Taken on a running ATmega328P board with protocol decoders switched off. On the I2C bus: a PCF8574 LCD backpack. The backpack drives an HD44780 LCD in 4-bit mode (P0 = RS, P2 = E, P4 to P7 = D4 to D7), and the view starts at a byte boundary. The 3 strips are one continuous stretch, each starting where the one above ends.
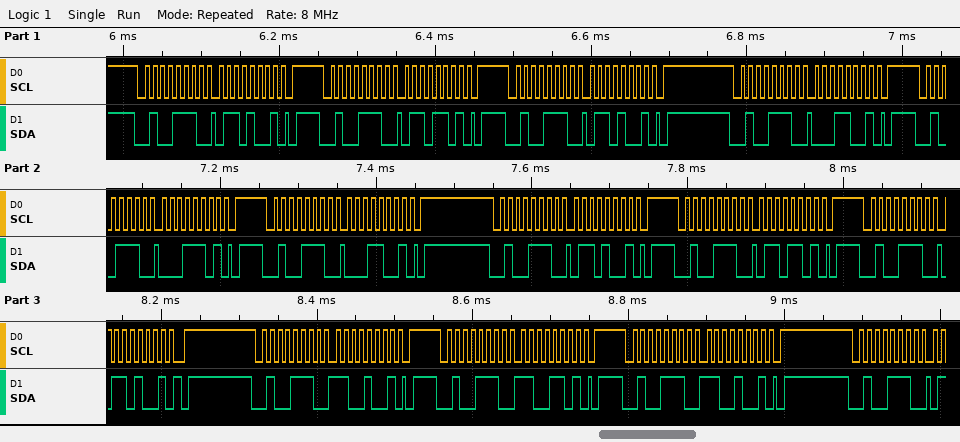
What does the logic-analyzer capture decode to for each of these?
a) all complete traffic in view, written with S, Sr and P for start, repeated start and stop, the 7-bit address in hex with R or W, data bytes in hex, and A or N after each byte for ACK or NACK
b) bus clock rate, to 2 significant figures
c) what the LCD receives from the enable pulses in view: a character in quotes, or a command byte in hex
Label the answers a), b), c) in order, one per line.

a) S 27W A 69 A P S 27W A 6D A P S 27W A 69 A P S 27W A 19 A P S 27W A 1D A P S 27W A 19 A P S 27W A 69 A P S 27W A 6D A P S 27W A 69 A P S 27W A C9 A P S 27W A CD A P S 27W A C9 A P S 27W A
b) 100 kHz
c) 'a' 'l'
